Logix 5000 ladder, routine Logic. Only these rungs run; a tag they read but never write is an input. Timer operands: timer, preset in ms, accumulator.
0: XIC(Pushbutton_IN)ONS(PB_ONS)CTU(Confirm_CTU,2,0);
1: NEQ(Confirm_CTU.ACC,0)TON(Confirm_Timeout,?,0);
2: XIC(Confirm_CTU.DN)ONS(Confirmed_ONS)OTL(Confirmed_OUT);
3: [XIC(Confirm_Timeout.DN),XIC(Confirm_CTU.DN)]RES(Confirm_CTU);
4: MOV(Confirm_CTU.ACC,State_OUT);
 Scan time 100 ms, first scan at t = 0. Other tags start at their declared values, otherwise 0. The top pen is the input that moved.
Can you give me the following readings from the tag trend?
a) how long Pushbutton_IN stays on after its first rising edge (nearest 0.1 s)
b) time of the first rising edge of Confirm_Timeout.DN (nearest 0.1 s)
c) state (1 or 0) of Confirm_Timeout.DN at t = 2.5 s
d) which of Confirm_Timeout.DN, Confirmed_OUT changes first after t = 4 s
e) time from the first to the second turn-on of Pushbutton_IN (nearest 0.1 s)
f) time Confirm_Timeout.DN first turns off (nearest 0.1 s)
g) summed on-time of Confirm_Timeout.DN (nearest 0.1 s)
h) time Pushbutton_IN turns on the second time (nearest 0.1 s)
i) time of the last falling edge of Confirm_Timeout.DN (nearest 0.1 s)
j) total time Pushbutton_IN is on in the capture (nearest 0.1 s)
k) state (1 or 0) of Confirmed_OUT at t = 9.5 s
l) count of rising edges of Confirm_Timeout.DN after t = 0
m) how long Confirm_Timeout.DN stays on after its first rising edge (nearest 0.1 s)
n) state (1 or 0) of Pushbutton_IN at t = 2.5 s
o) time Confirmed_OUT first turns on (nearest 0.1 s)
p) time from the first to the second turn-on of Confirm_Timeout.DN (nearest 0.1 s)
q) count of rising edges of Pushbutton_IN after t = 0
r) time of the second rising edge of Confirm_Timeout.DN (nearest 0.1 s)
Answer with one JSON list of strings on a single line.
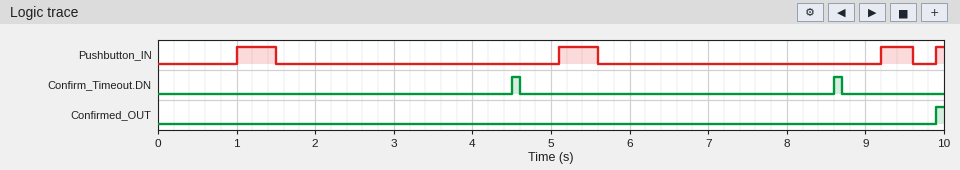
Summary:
["0.5 s", "4.5 s", "0", "Confirm_Timeout.DN", "4.1 s", "4.6 s", "0.2 s", "5.1 s", "8.7 s", "1.5 s", "0", "2", "0.1 s", "0", "9.9 s", "4.1 s", "4", "8.6 s"]
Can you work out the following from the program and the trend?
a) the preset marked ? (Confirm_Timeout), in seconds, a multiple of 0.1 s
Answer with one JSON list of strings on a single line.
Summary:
["3.5 s"]
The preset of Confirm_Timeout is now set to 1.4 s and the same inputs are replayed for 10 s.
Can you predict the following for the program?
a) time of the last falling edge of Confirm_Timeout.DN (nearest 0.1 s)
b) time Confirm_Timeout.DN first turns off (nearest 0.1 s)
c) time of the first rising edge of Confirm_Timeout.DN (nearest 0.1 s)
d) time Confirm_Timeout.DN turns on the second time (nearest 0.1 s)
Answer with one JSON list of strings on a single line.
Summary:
["6.6 s", "2.5 s", "2.4 s", "6.5 s"]
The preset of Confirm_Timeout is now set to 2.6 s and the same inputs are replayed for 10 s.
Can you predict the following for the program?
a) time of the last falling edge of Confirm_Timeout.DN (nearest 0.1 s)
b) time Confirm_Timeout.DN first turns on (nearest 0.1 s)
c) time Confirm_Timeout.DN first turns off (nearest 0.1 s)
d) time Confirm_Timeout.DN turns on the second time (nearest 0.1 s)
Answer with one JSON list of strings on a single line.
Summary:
["7.8 s", "3.6 s", "3.7 s", "7.7 s"]
